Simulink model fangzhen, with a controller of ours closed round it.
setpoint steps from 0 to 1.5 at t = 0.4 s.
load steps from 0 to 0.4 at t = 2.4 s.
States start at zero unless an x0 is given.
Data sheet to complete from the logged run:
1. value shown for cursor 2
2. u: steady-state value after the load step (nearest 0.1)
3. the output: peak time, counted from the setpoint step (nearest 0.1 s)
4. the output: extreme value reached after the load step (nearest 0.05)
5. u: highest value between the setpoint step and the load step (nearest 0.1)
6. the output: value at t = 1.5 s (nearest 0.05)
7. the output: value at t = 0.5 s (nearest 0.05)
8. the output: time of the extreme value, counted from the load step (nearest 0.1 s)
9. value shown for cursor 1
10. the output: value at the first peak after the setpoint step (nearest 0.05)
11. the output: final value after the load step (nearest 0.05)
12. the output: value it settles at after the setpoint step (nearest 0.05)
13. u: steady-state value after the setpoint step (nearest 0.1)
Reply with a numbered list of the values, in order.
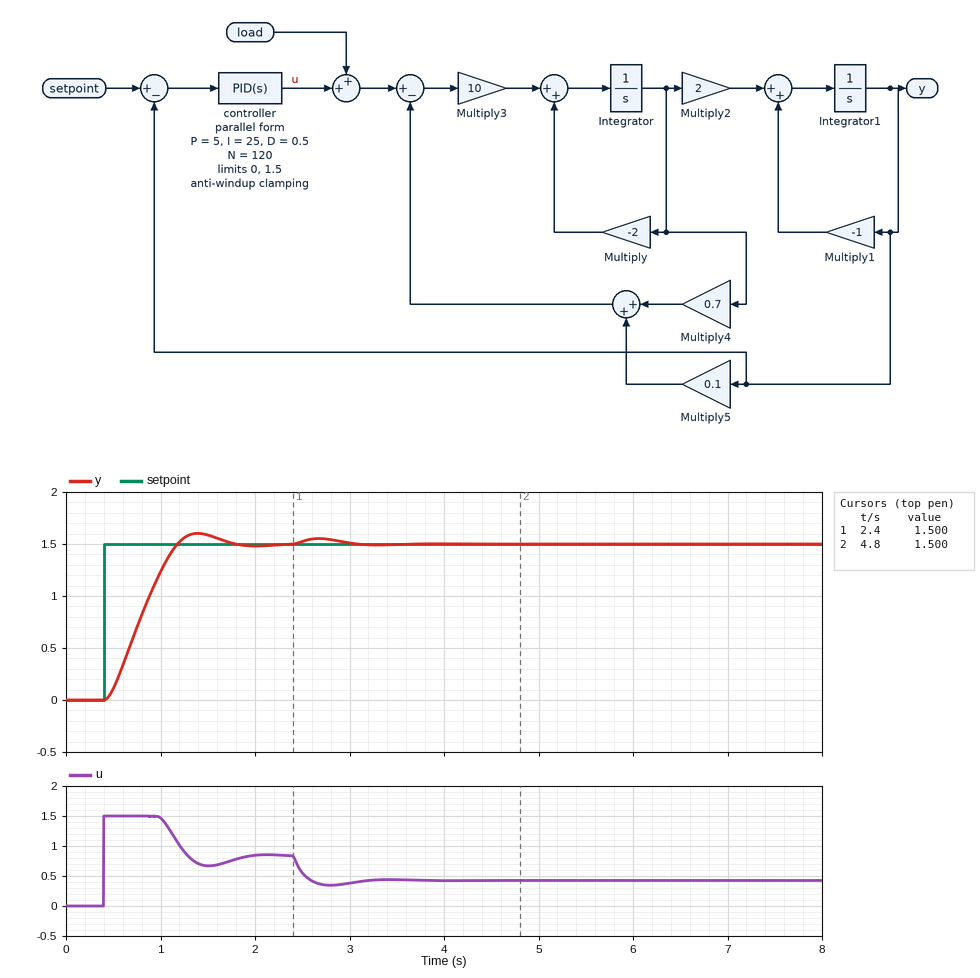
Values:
1. 1.500
2. 0.4
3. 1.0 s
4. 1.55
5. 1.5
6. 1.60
7. 0.10
8. 0.3 s
9. 1.500
10. 1.60
11. 1.50
12. 1.50
13. 0.8
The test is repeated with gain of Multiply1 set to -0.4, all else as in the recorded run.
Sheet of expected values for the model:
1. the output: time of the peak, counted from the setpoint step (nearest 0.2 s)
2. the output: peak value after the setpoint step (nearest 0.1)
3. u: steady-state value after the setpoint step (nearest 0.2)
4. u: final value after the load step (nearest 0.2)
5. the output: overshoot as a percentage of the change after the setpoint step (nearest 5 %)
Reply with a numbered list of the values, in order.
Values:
1. 0.8 s
2. 1.7
3. 0.4
4. 0.0
5. 10 %
